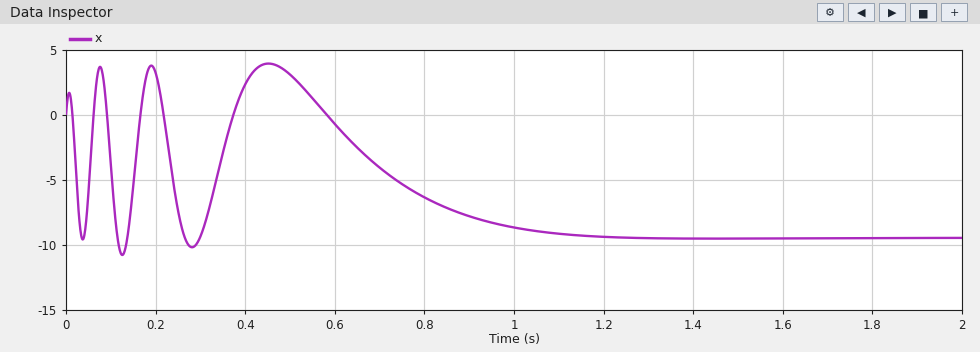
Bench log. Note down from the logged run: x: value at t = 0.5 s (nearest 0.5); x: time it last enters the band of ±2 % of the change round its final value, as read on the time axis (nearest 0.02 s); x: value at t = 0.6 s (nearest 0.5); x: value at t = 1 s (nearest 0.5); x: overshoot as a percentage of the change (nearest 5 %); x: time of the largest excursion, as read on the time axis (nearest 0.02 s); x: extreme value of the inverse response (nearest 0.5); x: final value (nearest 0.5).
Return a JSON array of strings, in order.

["3.0", "1.14 s", "-0.5", "-8.5", "15 %", "0.12 s", "4.0", "-9.5"]
